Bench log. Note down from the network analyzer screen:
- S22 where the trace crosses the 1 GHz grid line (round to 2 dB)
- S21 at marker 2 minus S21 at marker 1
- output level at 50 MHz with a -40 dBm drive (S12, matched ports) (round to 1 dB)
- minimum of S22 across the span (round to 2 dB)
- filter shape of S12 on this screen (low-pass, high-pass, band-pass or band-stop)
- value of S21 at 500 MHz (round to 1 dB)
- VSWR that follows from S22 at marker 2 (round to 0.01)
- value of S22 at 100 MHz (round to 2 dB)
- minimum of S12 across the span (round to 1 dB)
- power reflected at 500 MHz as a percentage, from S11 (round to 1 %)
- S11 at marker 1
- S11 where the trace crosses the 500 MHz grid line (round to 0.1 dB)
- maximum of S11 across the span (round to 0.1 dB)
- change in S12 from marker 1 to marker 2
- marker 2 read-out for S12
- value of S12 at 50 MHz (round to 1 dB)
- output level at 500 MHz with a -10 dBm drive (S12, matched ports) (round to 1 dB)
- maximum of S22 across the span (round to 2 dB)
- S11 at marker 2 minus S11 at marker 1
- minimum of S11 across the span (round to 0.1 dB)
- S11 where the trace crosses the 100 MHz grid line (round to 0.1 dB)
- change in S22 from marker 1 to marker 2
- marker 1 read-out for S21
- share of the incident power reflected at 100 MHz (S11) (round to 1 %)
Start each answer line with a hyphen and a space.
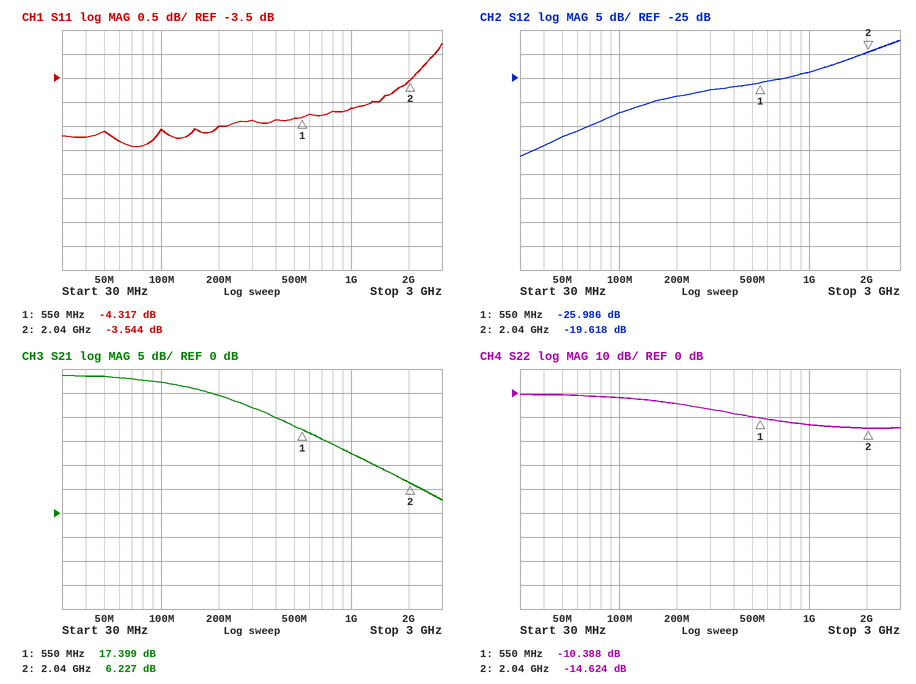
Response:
- -14 dB
- -11.172 dB
- -77 dBm
- -14 dB
- high-pass
- 18 dB
- 1.46
- -2 dB
- -41 dB
- 37 %
- -4.317 dB
- -4.3 dB
- -2.8 dB
- 6.368 dB
- -19.618 dB
- -37 dB
- -36 dBm
- 0 dB
- 0.773 dB
- -4.9 dB
- -4.6 dB
- -4.236 dB
- 17.399 dB
- 35 %
